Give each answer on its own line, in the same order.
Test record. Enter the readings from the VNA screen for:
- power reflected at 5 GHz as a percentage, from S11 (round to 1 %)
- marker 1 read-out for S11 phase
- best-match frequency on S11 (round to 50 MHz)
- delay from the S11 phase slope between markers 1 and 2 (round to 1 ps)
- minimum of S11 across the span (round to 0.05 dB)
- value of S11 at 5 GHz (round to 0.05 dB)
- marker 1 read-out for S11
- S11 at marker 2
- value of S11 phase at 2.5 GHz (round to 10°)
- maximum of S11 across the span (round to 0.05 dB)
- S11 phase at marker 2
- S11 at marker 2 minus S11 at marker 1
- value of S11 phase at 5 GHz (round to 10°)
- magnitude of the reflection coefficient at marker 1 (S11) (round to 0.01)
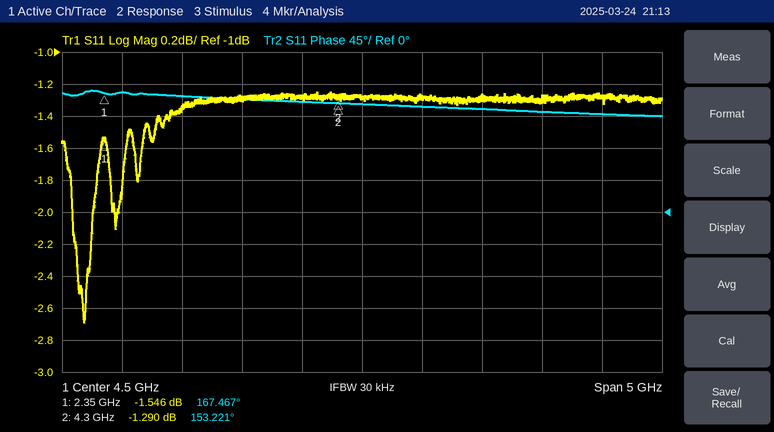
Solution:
74 %
167.467°
2.20 GHz
20 ps
-2.70 dB
-1.30 dB
-1.546 dB
-1.290 dB
170°
-1.25 dB
153.221°
0.256 dB
150°
0.84
